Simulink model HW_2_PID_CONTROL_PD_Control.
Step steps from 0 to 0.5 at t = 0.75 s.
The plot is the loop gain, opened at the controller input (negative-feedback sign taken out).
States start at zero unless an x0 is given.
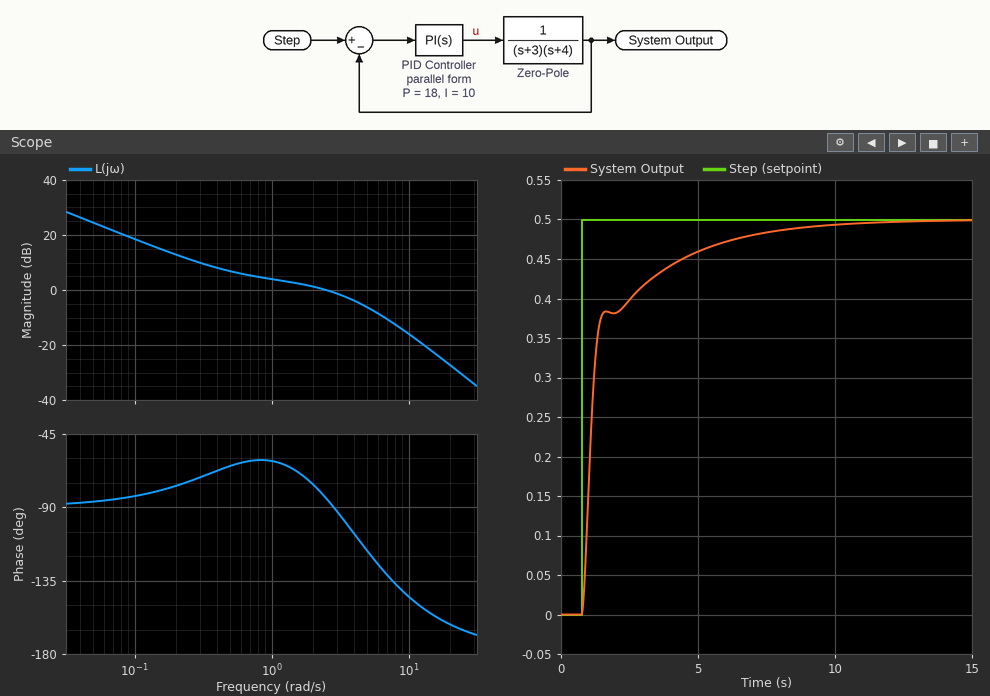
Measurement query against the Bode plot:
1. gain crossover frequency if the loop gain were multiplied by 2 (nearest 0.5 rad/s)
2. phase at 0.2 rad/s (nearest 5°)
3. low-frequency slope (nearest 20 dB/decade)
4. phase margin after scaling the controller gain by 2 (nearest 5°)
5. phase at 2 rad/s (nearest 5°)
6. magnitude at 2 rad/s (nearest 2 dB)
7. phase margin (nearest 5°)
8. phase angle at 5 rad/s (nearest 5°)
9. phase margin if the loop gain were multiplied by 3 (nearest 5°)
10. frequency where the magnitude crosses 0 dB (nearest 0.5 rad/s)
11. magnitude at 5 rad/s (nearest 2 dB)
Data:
5.0 rad/s
-75°
-20 dB/decade
65°
-75°
2 dB
95°
-115°
50°
2.5 rad/s
-6 dB
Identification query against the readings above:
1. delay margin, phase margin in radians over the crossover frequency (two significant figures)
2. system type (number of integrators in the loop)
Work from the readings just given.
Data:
0.66 s
1
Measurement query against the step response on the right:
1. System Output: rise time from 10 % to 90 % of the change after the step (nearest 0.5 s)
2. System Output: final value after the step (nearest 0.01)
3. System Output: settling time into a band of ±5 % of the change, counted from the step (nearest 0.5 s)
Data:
3.5 s
0.50
5.5 s
